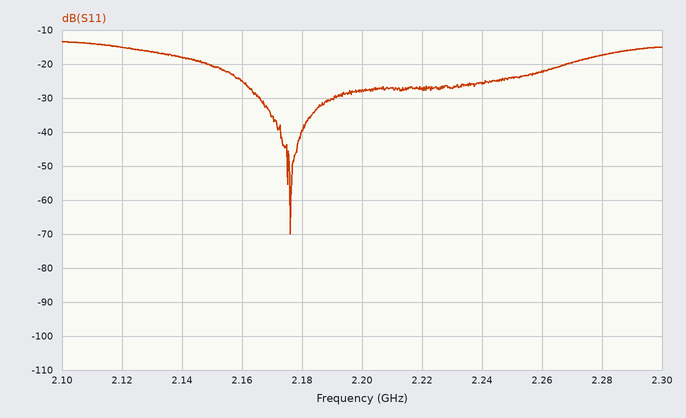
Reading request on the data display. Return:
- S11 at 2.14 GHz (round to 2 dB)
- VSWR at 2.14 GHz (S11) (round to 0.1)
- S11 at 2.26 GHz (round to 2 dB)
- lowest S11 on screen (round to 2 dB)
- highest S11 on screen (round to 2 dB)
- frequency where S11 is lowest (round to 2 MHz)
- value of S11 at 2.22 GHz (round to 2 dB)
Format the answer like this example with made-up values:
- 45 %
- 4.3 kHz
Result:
- -18 dB
- 1.3
- -22 dB
- -70 dB
- -14 dB
- 2.176 GHz
- -28 dB
